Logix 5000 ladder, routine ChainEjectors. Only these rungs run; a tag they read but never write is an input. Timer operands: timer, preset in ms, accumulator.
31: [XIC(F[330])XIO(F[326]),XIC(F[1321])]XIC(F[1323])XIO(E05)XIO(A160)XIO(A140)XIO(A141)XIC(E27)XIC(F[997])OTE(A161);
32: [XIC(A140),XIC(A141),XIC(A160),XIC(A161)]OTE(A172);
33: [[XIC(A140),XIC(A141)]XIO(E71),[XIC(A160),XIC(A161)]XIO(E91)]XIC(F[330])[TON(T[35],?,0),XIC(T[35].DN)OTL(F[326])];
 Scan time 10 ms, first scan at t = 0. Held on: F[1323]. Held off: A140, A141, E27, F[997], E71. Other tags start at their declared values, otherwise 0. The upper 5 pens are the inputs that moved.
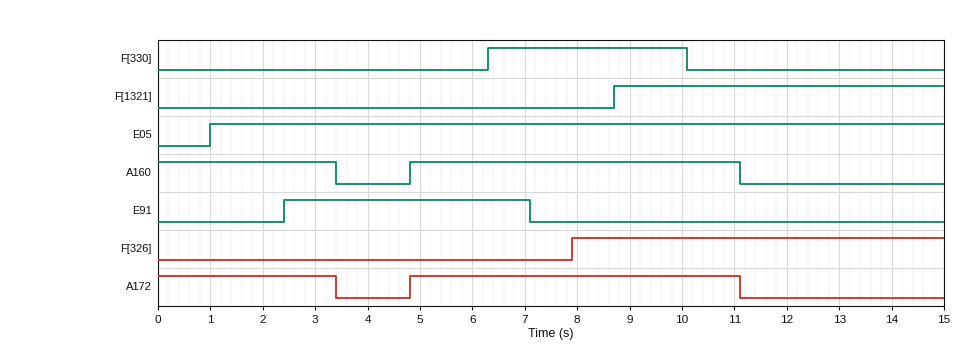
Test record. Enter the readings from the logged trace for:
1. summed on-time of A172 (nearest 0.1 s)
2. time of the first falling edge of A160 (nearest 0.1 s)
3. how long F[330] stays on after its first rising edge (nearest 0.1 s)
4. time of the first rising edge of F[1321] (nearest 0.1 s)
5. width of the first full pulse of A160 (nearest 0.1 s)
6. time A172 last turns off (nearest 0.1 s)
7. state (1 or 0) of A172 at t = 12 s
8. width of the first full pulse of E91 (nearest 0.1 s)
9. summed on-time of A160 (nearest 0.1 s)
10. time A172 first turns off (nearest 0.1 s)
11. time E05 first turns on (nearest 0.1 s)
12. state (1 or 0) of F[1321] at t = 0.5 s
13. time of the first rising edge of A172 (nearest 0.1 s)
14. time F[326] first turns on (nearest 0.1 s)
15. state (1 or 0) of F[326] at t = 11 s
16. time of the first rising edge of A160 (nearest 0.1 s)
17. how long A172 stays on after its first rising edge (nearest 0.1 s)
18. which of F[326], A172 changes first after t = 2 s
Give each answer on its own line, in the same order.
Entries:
9.7 s
3.4 s
3.8 s
8.7 s
6.3 s
11.1 s
0
4.7 s
9.7 s
3.4 s
1.0 s
0
4.8 s
7.9 s
1
4.8 s
6.3 s
A172
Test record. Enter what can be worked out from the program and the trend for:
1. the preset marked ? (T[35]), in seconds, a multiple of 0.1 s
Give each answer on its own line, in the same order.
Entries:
0.8 s
